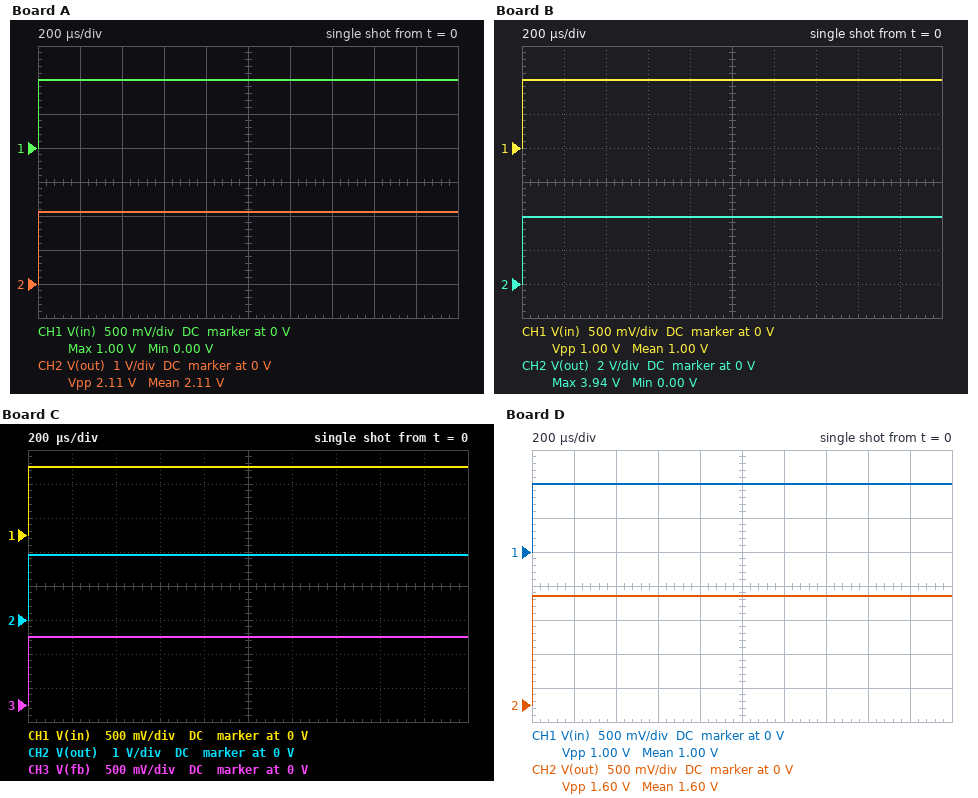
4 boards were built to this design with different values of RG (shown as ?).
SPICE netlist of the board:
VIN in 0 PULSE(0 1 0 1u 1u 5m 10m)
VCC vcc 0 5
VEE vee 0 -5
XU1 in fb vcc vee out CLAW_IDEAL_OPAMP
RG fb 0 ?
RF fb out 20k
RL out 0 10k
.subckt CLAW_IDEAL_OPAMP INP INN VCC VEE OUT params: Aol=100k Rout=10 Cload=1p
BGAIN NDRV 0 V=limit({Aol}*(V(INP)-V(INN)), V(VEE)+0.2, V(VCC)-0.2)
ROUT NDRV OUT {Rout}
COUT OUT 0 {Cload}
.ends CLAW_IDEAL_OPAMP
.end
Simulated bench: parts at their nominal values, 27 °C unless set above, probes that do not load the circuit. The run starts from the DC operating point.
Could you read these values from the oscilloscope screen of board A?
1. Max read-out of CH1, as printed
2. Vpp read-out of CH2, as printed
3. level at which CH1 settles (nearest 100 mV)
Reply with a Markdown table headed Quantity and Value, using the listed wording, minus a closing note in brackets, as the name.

| Quantity | Value |
|---|---|
| Max read-out of CH1, as printed | 1.00 V |
| Vpp read-out of CH2, as printed | 2.11 V |
| level at which CH1 settles | 1.0 V |
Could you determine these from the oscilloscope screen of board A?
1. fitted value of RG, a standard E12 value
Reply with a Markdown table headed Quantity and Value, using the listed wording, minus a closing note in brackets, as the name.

| Quantity | Value |
|---|---|
| fitted value of RG, a standard E12 value | 18 kΩ |
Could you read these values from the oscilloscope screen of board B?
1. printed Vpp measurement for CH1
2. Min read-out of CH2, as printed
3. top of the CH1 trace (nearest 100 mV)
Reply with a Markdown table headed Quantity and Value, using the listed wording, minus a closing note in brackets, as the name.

| Quantity | Value |
|---|---|
| printed Vpp measurement for CH1 | 1.00 V |
| Min read-out of CH2, as printed | 0.00 V |
| top of the CH1 trace | 1.0 V |
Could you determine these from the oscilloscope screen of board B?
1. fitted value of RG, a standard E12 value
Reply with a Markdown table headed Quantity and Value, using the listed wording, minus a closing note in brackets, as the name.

| Quantity | Value |
|---|---|
| fitted value of RG, a standard E12 value | 6.8 kΩ |
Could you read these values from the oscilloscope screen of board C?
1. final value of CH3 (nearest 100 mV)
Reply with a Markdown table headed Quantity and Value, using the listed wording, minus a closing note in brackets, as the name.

| Quantity | Value |
|---|---|
| final value of CH3 | 1.0 V |
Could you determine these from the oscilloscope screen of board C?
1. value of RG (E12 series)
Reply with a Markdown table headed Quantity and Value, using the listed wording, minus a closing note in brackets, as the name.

| Quantity | Value |
|---|---|
| value of RG | 22 kΩ |
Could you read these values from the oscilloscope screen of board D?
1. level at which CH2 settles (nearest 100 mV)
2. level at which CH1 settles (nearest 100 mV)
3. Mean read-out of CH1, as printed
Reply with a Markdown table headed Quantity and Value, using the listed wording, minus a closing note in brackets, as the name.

| Quantity | Value |
|---|---|
| level at which CH2 settles | 1.6 V |
| level at which CH1 settles | 1.0 V |
| Mean read-out of CH1, as printed | 1.00 V |
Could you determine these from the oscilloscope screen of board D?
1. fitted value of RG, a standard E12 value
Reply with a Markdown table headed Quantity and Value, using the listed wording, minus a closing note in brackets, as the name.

| Quantity | Value |
|---|---|
| fitted value of RG, a standard E12 value | 33 kΩ |
